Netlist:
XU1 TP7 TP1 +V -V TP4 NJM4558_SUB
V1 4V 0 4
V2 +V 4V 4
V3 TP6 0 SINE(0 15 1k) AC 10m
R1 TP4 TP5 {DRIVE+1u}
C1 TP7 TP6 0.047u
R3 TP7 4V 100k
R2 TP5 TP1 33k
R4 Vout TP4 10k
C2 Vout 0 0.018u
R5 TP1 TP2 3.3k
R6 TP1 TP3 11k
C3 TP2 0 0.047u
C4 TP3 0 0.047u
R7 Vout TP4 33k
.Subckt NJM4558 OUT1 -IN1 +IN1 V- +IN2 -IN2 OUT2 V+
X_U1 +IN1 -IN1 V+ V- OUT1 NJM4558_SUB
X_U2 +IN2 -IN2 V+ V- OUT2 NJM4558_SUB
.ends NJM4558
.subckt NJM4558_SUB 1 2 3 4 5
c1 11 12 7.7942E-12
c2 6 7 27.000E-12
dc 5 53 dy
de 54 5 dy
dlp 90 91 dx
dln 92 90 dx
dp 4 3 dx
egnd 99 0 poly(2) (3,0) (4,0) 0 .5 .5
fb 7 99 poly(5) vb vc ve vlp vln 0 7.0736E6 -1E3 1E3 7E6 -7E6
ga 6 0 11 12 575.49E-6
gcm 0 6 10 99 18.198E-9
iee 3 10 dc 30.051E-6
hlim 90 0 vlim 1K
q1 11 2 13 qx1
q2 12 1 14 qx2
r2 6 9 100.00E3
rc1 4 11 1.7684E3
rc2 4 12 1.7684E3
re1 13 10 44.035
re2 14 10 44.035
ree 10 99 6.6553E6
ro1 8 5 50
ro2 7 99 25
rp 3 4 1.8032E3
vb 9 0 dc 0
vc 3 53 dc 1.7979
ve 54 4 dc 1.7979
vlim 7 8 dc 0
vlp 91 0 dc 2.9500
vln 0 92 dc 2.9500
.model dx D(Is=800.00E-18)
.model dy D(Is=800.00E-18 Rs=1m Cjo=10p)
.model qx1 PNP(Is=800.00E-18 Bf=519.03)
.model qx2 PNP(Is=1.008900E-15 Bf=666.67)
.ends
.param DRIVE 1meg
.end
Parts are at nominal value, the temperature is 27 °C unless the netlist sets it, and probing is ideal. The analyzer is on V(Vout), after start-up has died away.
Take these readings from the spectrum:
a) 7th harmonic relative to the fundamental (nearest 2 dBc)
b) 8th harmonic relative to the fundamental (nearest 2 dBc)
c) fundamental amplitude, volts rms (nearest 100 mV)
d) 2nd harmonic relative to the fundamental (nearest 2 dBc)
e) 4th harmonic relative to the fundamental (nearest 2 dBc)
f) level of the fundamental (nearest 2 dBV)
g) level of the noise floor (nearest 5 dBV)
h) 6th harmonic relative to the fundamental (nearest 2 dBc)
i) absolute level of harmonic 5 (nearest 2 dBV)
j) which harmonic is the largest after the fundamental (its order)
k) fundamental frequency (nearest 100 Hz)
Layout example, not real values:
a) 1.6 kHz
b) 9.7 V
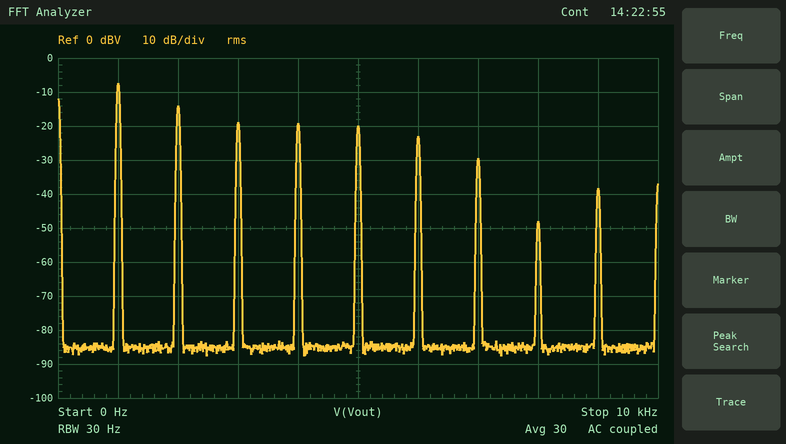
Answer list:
a) -22 dBc
b) -40 dBc
c) 400 mV
d) -6 dBc
e) -12 dBc
f) -8 dBV
g) -85 dBV
h) -16 dBc
i) -20 dBV
j) 2
k) 1.0 kHz
